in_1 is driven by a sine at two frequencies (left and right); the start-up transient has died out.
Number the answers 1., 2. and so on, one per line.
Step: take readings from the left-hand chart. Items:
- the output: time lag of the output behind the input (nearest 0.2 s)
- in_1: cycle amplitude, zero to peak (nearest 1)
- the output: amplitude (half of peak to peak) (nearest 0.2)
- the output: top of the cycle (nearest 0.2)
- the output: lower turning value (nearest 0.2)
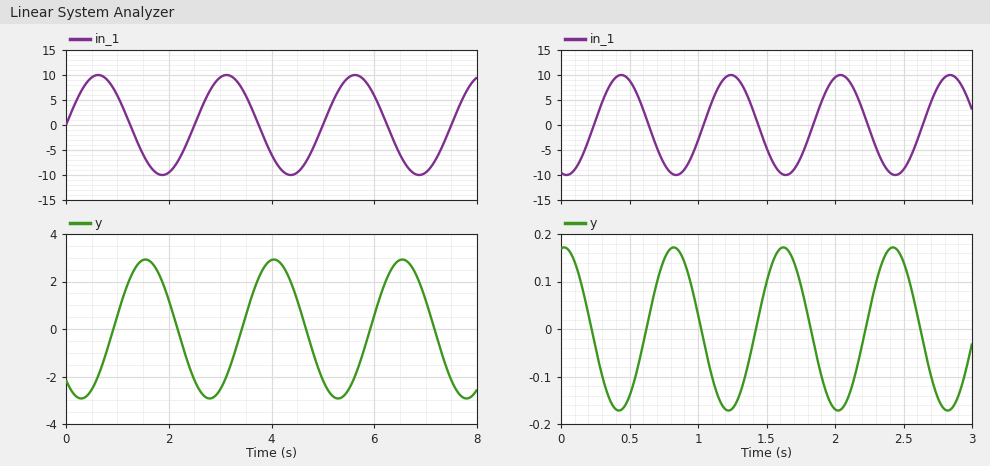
1. 1.0 s
2. 10
3. 3.0
4. 3.0
5. -3.0
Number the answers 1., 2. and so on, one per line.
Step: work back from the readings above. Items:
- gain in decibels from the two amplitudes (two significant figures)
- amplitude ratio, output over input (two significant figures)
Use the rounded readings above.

1. -10 dB
2. 0.30
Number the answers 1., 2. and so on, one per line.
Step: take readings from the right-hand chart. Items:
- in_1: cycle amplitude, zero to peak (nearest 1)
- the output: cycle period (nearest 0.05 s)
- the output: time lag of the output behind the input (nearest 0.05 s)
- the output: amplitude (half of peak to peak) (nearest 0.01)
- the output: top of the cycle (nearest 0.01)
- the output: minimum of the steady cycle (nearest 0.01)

1. 10
2. 0.80 s
3. 0.40 s
4. 0.17
5. 0.17
6. -0.17
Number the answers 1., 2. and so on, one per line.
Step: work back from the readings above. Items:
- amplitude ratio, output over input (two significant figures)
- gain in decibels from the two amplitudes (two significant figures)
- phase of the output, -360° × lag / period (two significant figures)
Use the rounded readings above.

1. 0.017
2. -35 dB
3. -180°
